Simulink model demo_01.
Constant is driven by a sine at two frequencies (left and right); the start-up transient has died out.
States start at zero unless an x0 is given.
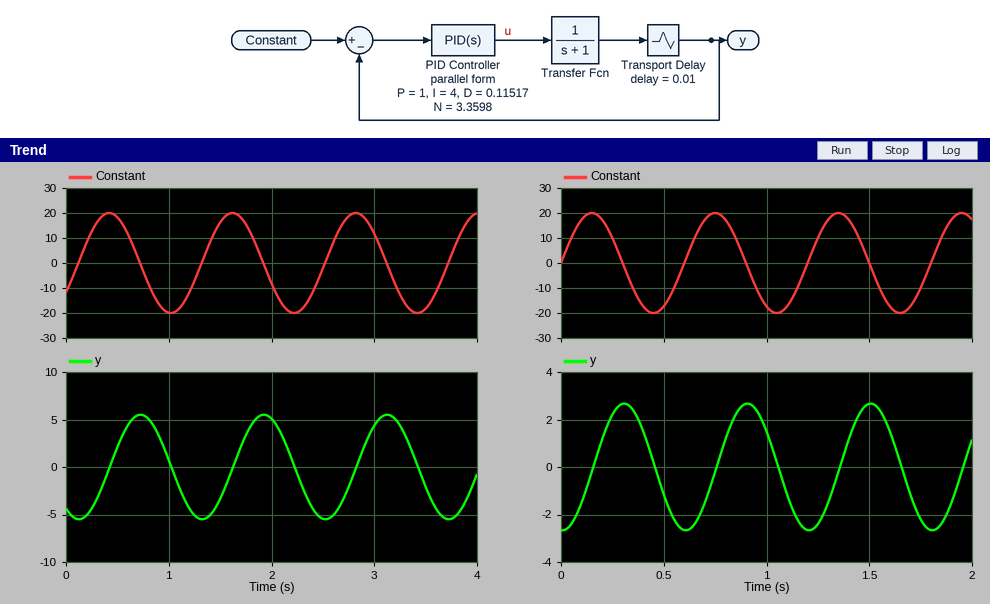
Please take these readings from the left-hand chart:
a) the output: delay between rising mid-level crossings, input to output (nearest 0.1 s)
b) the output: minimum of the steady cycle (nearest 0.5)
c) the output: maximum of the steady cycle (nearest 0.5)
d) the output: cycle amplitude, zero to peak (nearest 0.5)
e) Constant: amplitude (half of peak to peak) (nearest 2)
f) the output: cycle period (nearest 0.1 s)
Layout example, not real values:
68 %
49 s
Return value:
0.3 s
-5.5
5.5
5.5
20
1.2 s
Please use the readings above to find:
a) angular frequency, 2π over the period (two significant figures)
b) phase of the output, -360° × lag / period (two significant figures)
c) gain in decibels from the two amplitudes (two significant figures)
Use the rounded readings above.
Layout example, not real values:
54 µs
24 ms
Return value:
5.2 rad/s
-90°
-11 dB
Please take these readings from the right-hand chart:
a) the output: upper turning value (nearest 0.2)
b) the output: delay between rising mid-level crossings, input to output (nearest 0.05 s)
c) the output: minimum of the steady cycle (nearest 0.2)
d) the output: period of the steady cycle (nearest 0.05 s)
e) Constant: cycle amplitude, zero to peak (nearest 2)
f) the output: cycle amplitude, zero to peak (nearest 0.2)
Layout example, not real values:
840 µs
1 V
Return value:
2.6
0.15 s
-2.6
0.60 s
20
2.6
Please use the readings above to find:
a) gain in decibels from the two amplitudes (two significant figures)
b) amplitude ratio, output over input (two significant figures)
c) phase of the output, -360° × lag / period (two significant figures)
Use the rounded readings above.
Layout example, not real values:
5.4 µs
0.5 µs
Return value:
-18 dB
0.13
-90°
